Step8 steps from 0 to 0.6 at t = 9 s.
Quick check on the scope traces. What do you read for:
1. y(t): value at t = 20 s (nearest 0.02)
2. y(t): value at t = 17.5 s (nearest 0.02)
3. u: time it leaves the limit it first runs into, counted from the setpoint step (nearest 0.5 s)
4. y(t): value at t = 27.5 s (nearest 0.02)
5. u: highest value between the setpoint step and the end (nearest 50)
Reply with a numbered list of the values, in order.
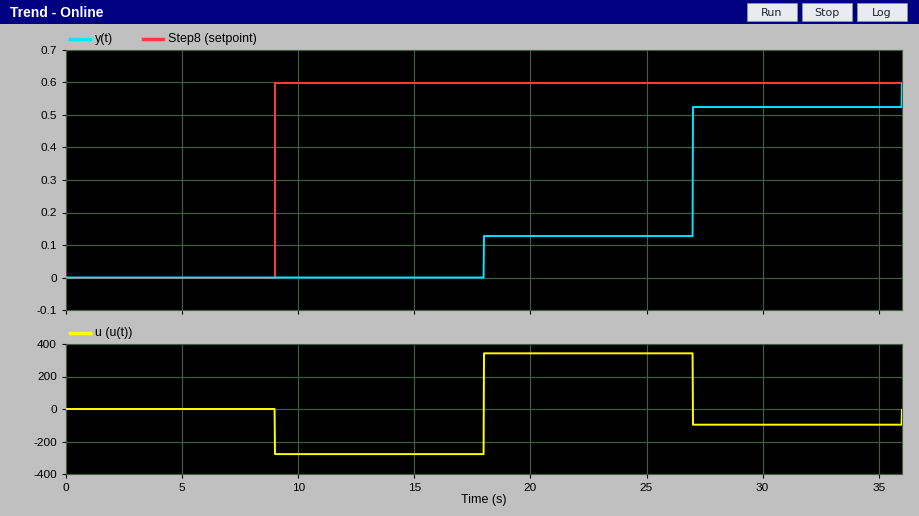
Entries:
1. 0.12
2. 0.00
3. 9.0 s
4. 0.52
5. 350
